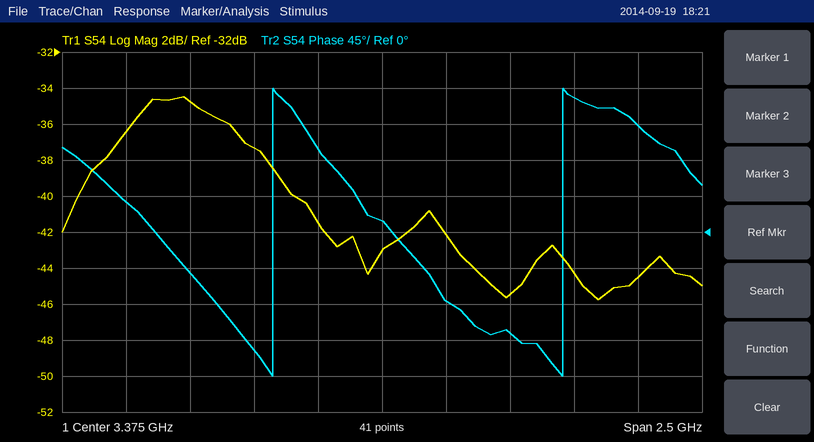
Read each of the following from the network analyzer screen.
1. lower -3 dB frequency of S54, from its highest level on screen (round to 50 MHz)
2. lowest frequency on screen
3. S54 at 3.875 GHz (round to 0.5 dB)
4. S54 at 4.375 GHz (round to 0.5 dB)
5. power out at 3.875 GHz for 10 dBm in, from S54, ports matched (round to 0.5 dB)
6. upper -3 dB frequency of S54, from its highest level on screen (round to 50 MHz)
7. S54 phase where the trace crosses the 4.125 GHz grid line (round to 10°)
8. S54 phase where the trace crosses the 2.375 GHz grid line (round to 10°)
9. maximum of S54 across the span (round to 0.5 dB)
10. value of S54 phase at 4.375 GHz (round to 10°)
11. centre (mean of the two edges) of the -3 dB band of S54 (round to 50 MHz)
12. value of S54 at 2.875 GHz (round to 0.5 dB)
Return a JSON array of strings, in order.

["2.30 GHz", "2.125 GHz", "-45.5 dB", "-44.5 dB", "-35.5 dBm", "2.90 GHz", "170°", "40°", "-34.5 dB", "130°", "2.60 GHz", "-37.5 dB"]
